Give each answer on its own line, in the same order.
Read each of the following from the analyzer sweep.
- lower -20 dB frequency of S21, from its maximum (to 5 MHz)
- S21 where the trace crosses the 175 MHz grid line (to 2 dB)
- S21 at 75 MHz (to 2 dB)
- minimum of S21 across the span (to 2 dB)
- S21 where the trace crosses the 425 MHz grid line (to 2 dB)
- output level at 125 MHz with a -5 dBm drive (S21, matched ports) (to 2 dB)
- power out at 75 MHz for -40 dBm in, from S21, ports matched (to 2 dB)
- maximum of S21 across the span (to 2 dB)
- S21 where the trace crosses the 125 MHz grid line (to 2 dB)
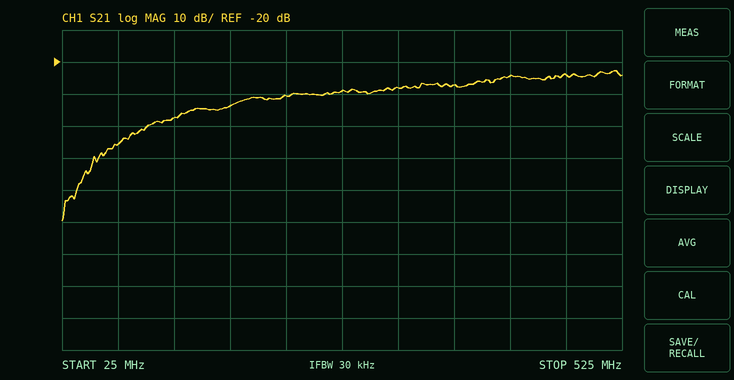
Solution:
85 MHz
-34 dB
-46 dB
-70 dB
-24 dB
-42 dBm
-86 dBm
-22 dB
-38 dB
